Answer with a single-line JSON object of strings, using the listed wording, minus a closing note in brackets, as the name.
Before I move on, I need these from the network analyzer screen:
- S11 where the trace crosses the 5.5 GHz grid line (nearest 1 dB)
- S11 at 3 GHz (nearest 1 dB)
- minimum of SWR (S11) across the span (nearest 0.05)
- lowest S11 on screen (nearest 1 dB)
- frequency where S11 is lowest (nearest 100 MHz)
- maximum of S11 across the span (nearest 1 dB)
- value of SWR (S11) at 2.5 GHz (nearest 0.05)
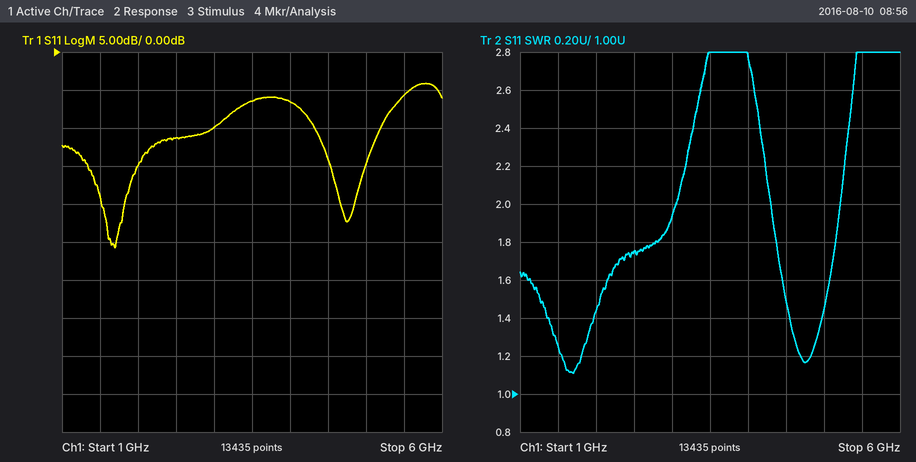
{"S11 where the trace crosses the 5.5 GHz grid line": "-6 dB", "S11 at 3 GHz": "-10 dB", "minimum of SWR (S11) across the span": "1.10", "lowest S11 on screen": "-26 dB", "frequency where S11 is lowest": "1.7 GHz", "maximum of S11 across the span": "-4 dB", "value of SWR (S11) at 2.5 GHz": "1.75"}
